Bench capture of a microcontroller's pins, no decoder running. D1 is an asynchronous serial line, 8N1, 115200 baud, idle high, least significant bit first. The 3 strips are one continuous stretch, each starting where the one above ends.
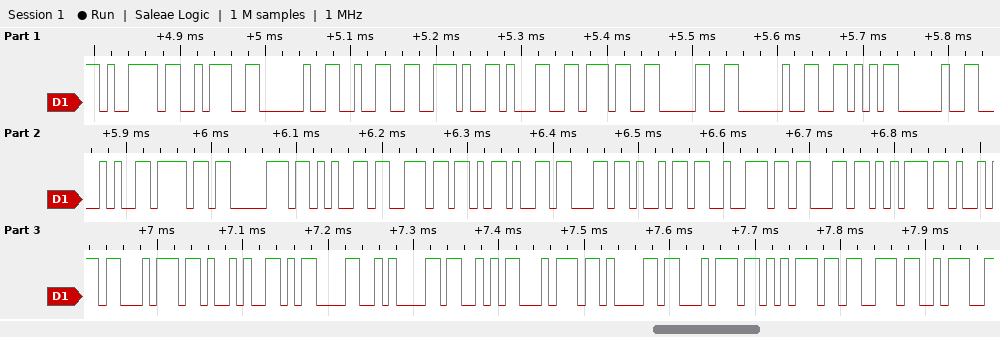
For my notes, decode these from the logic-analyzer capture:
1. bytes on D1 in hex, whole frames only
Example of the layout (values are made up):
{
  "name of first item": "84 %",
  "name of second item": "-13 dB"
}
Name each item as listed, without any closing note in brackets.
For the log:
{
  "bytes on D1 in hex, whole frames only": "0x79 0x3A 0x20 0x32 0x2E 0x31 0x37 0x30 0x20 0x56 0x20 0x28 0x6F 0x70 0x65 0x6E 0x2D 0x63 0x69 0x72 0x63 0x75 0x69 0x74 0x29 0x0D 0x0A 0x53 0x74 0x61 0x74 0x75 0x73 0x3A"
}
